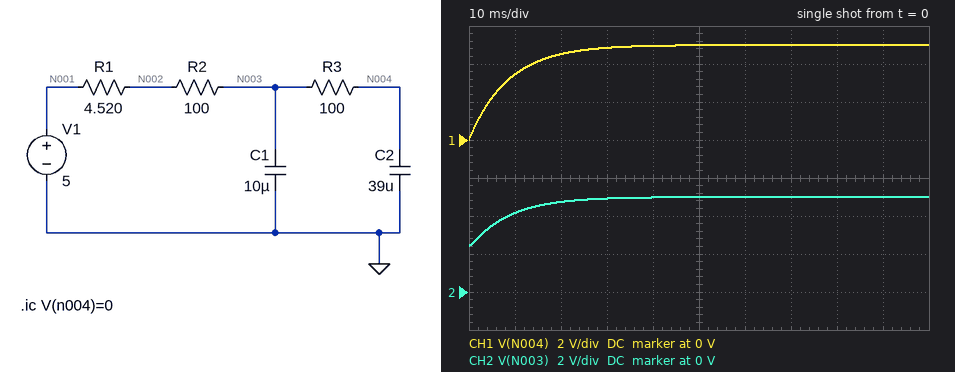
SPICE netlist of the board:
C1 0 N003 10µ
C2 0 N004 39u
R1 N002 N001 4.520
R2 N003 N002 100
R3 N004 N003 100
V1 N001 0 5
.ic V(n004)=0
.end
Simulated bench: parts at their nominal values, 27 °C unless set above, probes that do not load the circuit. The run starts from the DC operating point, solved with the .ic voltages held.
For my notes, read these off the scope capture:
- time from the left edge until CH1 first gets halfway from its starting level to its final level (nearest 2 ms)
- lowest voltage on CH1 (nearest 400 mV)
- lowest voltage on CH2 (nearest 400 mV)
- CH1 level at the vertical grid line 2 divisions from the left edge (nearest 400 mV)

6 ms
0 V
2.4 V
4.4 V
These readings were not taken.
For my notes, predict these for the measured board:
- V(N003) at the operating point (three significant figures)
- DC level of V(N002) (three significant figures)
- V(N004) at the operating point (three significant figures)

5.00 V
5.00 V
5.00 V
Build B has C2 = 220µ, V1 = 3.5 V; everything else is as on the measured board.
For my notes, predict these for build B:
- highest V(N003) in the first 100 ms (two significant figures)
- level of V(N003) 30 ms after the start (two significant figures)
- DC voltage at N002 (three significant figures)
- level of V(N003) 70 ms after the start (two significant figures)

3.3 V
2.6 V
3.50 V
3.1 V
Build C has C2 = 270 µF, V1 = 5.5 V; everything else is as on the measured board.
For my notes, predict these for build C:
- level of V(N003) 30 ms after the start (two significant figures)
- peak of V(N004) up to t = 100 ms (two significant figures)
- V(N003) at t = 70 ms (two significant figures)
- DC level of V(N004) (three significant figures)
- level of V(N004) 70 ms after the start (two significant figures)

3.8 V
4.6 V
4.7 V
5.50 V
3.9 V
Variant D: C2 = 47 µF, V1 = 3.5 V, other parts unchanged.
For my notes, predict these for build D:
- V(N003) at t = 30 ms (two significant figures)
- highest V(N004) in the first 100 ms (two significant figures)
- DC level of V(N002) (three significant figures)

3.4 V
3.5 V
3.50 V
